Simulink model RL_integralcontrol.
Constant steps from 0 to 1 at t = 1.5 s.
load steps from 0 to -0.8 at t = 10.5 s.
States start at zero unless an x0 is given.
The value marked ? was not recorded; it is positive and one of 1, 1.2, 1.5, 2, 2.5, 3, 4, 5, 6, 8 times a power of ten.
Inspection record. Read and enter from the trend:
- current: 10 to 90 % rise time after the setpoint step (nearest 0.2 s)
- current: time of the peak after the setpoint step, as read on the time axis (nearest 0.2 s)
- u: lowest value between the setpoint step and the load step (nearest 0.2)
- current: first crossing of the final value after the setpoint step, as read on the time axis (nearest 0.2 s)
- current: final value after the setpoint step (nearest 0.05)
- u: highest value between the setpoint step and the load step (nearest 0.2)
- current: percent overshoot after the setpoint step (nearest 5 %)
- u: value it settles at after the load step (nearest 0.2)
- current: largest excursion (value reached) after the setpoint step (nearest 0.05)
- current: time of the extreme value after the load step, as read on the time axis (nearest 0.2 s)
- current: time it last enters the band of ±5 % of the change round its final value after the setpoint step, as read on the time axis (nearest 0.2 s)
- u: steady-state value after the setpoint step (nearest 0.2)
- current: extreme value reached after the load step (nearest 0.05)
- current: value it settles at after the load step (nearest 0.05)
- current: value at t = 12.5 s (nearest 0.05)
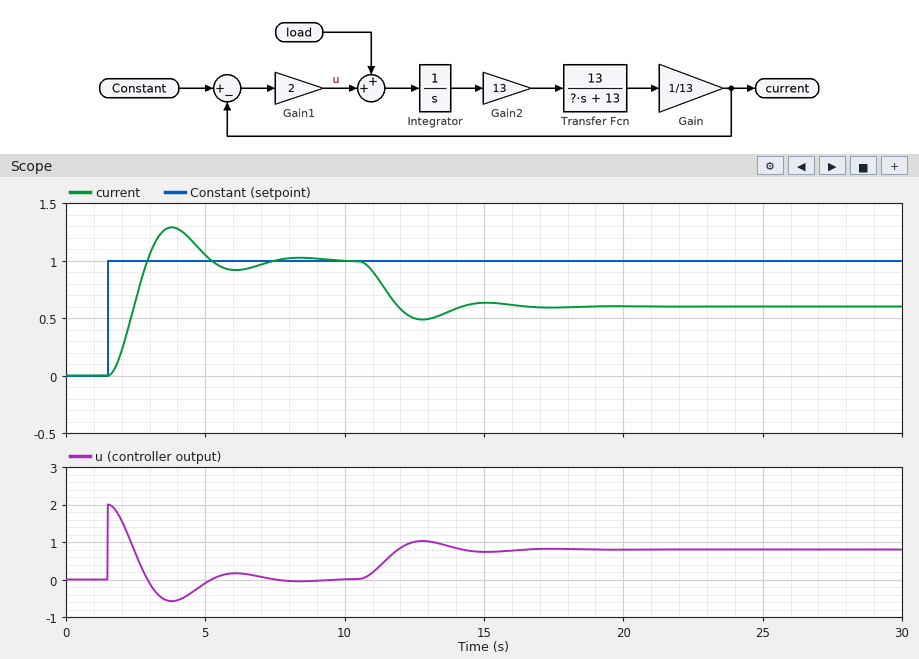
1.0 s
3.8 s
-0.6
3.0 s
1.00
2.0
30 %
0.8
1.30
12.8 s
6.8 s
0.0
0.50
0.60
0.50
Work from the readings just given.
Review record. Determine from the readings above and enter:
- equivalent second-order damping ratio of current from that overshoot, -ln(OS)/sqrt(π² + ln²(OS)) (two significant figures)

0.36
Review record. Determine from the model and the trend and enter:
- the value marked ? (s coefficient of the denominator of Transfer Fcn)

12
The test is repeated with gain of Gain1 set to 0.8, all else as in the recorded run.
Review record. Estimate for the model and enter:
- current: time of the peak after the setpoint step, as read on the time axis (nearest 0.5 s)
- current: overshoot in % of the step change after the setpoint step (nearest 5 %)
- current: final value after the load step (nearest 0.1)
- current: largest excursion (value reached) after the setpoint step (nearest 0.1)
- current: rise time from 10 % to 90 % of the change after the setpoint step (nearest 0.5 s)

5.5 s
10 %
0.0
1.1
2.0 s
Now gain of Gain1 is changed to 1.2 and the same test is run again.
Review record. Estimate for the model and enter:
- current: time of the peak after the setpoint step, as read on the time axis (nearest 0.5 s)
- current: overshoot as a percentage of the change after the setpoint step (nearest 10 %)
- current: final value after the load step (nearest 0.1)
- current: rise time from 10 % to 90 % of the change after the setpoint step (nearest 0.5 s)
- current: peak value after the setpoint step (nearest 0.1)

4.5 s
20 %
0.3
1.5 s
1.2
